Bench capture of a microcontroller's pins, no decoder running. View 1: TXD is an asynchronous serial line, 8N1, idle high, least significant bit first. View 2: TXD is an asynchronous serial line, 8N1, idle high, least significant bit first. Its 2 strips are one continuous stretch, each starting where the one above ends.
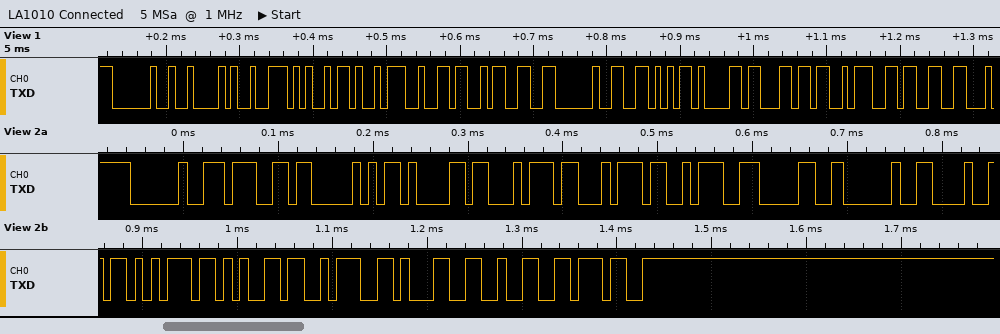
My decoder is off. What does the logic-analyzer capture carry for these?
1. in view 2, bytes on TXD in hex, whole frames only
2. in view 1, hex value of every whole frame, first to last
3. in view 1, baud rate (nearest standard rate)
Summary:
20 67 50 61 74 74 3A 30 20 48 75 65 3A 31 32 37
0x20 0x42 0x72 0x69 0x3A 0x36 0x33 0x20 0x56 0x61 0x6C 0x3A 0x33
115200 baud
